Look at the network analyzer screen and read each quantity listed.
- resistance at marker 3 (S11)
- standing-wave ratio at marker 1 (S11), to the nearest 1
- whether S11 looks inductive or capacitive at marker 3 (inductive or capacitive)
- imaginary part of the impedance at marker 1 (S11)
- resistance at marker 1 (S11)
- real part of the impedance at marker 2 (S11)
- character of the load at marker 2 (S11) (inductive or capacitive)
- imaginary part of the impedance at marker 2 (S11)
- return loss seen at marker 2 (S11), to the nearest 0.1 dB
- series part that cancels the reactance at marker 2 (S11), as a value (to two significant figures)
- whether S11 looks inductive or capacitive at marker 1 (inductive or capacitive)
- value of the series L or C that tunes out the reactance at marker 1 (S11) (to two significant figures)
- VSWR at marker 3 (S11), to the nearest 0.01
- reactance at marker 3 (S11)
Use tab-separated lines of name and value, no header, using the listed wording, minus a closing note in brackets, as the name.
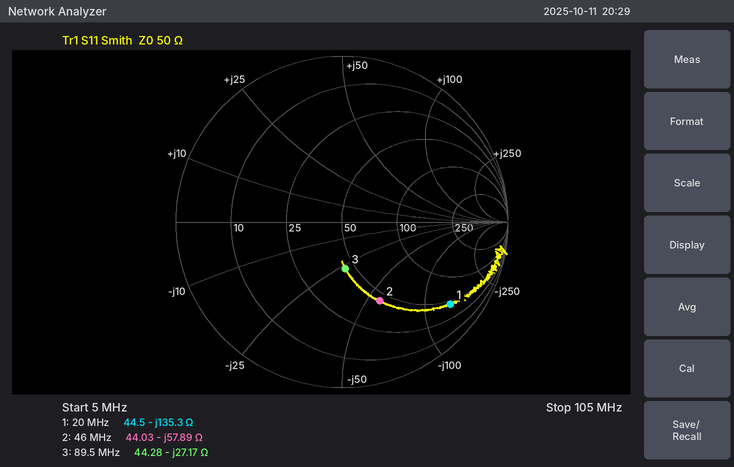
resistance at marker 3	44.28 Ω
standing-wave ratio at marker 1 (S11), to the nearest 1	10
whether S11 looks inductive or capacitive at marker 3	capacitive
imaginary part of the impedance at marker 1	-135.3 Ω
resistance at marker 1	44.5 Ω
real part of the impedance at marker 2	44.03 Ω
character of the load at marker 2 (S11)	capacitive
imaginary part of the impedance at marker 2	-57.89 Ω
return loss seen at marker 2 (S11), to the nearest 0.1 dB	5.6 dB
series part that cancels the reactance at marker 2 (S11), as a value	200 nH
whether S11 looks inductive or capacitive at marker 1	capacitive
value of the series L or C that tunes out the reactance at marker 1 (S11)	1.1 µH
VSWR at marker 3 (S11), to the nearest 0.01	1.79
reactance at marker 3	-27.17 Ω
